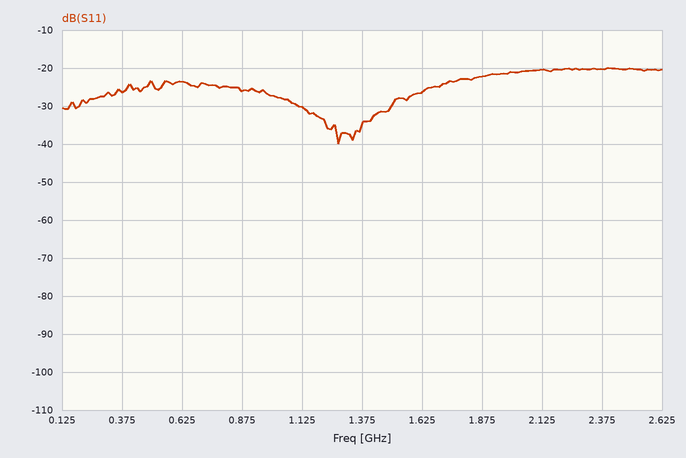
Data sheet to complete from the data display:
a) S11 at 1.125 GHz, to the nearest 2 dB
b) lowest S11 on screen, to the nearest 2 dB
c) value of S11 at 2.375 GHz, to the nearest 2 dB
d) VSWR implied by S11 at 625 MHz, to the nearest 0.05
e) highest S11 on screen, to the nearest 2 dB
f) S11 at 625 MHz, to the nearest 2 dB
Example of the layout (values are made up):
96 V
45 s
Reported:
-30 dB
-40 dB
-20 dB
1.15
-20 dB
-24 dB
